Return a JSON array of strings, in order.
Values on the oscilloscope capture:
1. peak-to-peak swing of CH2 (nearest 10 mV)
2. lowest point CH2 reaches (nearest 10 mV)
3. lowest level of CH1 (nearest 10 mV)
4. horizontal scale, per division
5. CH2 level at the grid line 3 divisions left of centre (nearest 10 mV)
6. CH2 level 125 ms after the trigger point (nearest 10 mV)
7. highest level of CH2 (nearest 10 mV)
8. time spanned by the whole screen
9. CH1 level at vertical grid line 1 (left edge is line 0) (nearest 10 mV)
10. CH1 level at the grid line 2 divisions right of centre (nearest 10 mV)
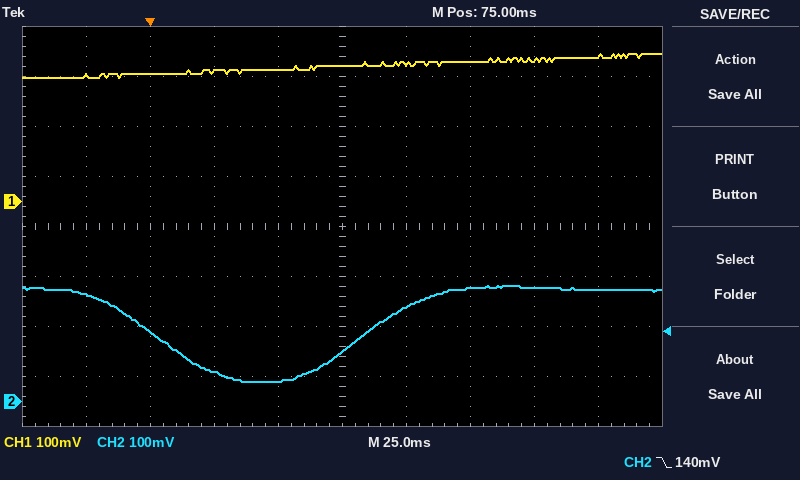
["190 mV", "40 mV", "250 mV", "25 ms", "140 mV", "230 mV", "230 mV", "250 ms", "250 mV", "280 mV"]
